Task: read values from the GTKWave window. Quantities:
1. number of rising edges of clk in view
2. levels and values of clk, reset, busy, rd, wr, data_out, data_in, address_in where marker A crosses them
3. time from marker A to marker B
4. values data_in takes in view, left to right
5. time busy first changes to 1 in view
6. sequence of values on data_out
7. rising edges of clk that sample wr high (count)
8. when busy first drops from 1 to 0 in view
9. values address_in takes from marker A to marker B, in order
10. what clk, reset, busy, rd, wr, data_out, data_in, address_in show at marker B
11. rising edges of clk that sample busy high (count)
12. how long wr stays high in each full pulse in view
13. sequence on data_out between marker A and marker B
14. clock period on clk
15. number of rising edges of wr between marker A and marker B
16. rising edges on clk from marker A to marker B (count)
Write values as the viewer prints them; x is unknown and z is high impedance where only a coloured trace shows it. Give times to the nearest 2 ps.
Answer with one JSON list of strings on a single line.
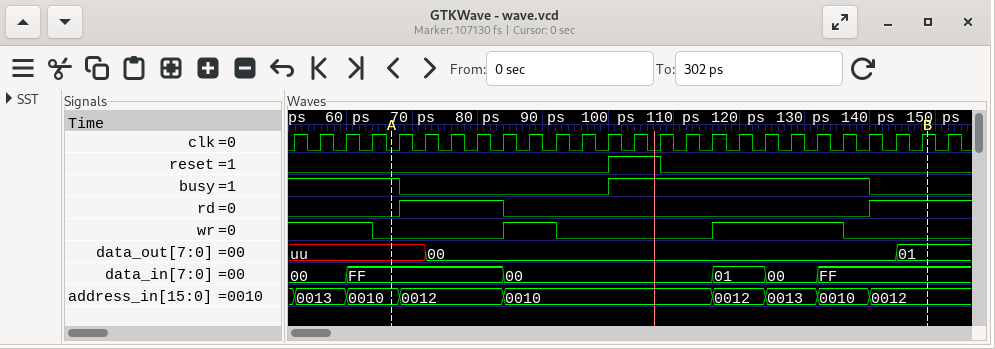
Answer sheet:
["26", "clk=0, reset=0, busy=1, rd=0, wr=0, data_out=uu, data_in=FF, address_in=0010", "82 ps", "00, FF, 00, 01, 00, FF", "100 ps", "uu, 00, 01", "11", "68 ps", "0010, 0012, 0010, 0012, 0013, 0010, 0012", "clk=1, reset=0, busy=0, rd=1, wr=0, data_out=01, data_in=FF, address_in=0012", "15", "8 ps, 20 ps", "uu, 00, 01", "4 ps", "2", "21"]
